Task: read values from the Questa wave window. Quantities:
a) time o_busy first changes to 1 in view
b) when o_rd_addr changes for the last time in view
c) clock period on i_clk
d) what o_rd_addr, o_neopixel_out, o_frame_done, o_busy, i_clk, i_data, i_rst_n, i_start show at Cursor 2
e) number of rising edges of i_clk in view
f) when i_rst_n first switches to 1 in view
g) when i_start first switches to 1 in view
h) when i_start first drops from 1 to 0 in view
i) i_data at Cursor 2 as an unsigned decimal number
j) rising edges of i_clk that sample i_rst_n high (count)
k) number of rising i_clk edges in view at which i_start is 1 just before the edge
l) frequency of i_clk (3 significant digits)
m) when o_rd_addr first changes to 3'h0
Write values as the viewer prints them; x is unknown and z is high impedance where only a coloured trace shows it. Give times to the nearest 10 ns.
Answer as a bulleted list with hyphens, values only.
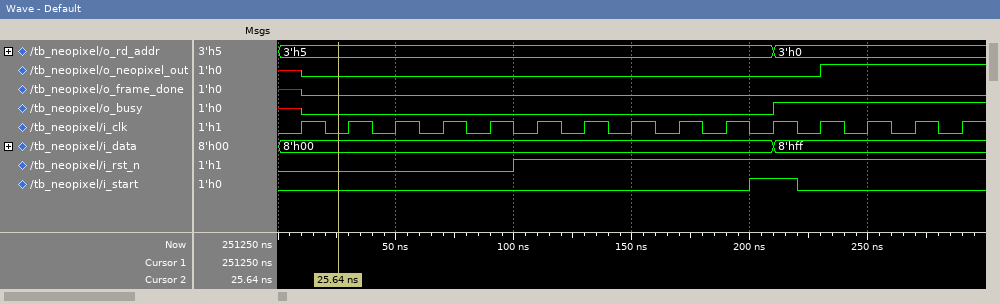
- 210 ns
- 210 ns
- 20 ns
- o_rd_addr=3'h5, o_neopixel_out=0, o_frame_done=0, o_busy=0, i_clk=0, i_data=8'h00, i_rst_n=0, i_start=0
- 15
- 100 ns
- 200 ns
- 220 ns
- 0
- 10
- 1
- 50.0 MHz
- 210 ns
